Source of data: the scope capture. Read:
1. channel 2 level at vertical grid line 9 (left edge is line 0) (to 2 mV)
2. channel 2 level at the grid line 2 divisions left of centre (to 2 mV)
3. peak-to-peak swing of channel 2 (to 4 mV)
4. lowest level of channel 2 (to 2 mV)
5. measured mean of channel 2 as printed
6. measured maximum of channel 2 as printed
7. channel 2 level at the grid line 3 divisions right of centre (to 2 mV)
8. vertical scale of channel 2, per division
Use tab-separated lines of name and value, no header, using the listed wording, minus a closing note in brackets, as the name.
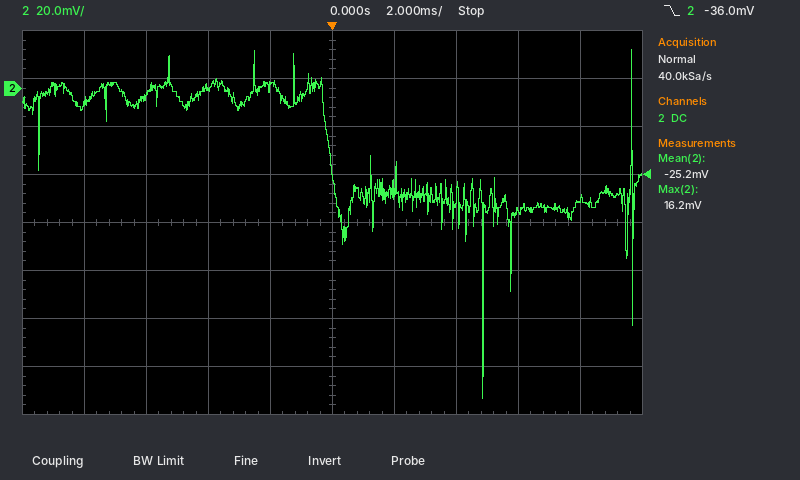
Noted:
channel 2 level at vertical grid line 9 (left edge is line 0)	-46 mV
channel 2 level at the grid line 2 divisions left of centre	0 mV
peak-to-peak swing of channel 2	144 mV
lowest level of channel 2	-130 mV
measured mean of channel 2 as printed	-25.2 mV
measured maximum of channel 2 as printed	16.2 mV
channel 2 level at the grid line 3 divisions right of centre	-52 mV
vertical scale of channel 2, per division	20 mV
